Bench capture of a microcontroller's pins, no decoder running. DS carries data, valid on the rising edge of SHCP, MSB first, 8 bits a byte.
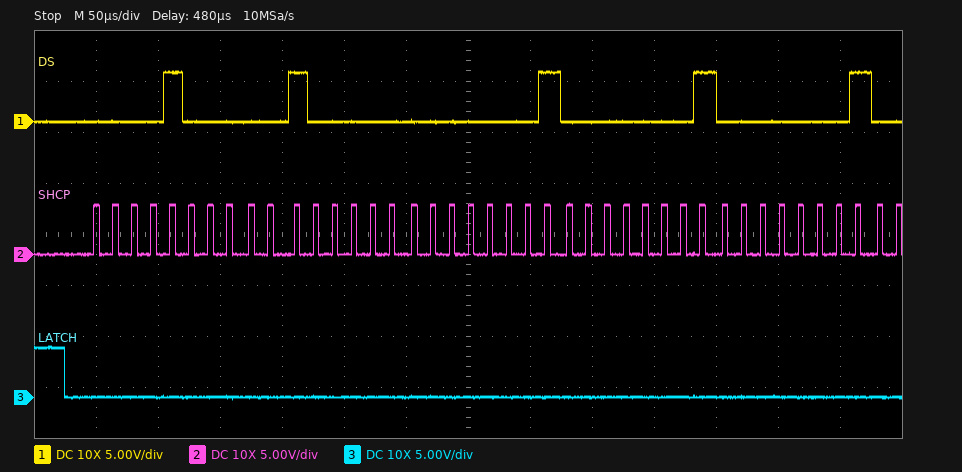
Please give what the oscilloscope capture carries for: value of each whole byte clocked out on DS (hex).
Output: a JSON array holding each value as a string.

["0x08 0x20 0x01 0x01 0x01"]
